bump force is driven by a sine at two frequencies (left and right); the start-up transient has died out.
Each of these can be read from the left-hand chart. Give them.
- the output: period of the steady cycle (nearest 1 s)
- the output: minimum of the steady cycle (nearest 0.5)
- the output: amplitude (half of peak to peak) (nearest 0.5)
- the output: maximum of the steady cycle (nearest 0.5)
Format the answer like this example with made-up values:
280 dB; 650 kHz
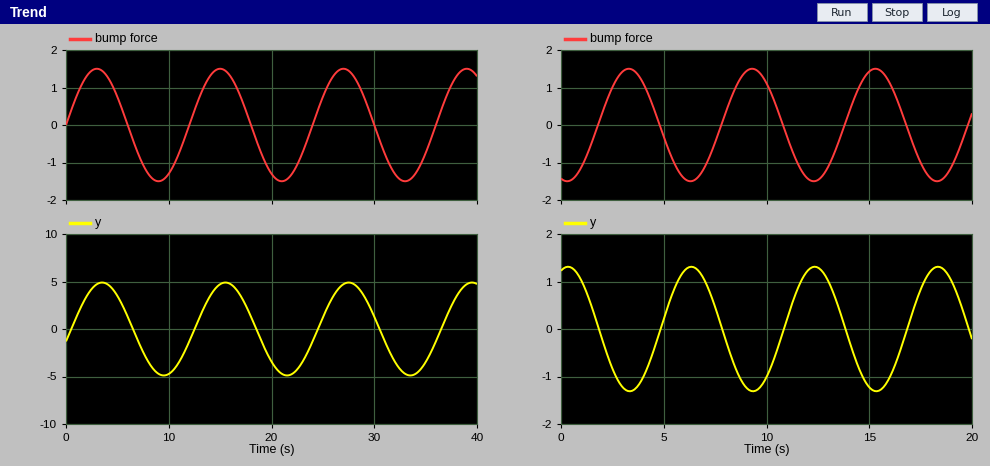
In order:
12 s; -5.0; 5.0; 5.0
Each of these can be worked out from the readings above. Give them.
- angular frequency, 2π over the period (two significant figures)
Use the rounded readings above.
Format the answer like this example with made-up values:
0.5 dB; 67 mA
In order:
0.52 rad/s
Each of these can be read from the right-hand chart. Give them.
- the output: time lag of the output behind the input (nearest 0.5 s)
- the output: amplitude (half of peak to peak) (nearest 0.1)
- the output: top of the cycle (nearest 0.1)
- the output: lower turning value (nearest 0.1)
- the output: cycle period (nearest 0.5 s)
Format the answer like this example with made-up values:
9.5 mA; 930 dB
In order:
3.0 s; 1.3; 1.3; -1.3; 6.0 s
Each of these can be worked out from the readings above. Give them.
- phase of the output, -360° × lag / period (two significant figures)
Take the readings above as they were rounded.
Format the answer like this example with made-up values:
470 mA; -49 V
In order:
-180°
